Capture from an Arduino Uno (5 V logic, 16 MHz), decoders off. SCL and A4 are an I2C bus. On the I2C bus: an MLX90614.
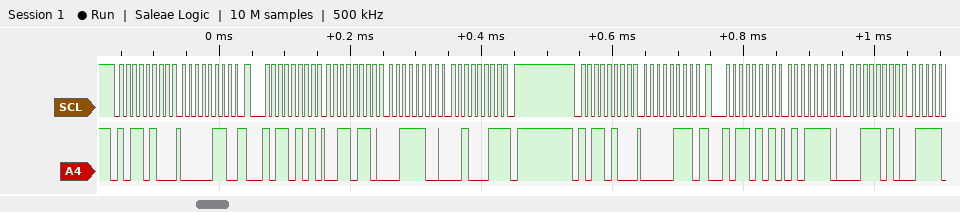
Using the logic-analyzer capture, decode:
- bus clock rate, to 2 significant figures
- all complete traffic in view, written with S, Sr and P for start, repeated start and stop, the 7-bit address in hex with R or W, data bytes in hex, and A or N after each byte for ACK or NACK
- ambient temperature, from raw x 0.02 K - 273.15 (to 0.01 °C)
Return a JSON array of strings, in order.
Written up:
["100 kHz", "S 5AW A 06 A Sr 5AR A 36 A 3C A 23 N P S 5AW A 07 A Sr 5AR A 5E A 3A A", "35.13 °C"]
